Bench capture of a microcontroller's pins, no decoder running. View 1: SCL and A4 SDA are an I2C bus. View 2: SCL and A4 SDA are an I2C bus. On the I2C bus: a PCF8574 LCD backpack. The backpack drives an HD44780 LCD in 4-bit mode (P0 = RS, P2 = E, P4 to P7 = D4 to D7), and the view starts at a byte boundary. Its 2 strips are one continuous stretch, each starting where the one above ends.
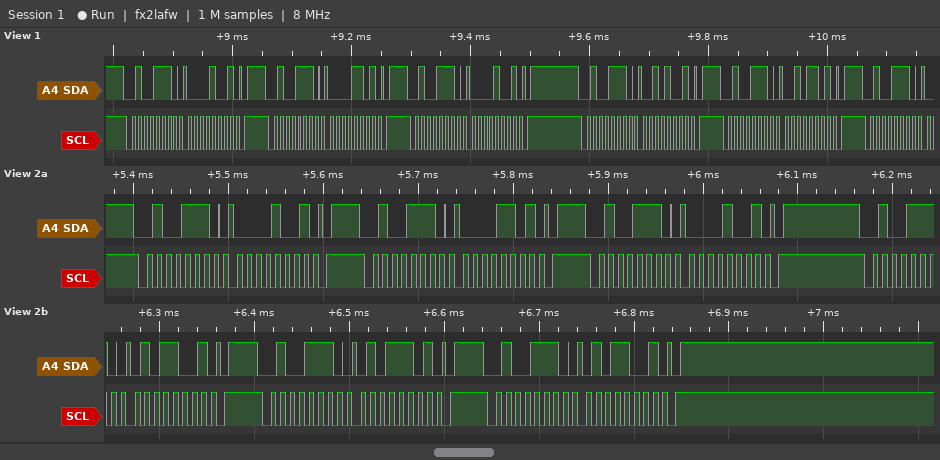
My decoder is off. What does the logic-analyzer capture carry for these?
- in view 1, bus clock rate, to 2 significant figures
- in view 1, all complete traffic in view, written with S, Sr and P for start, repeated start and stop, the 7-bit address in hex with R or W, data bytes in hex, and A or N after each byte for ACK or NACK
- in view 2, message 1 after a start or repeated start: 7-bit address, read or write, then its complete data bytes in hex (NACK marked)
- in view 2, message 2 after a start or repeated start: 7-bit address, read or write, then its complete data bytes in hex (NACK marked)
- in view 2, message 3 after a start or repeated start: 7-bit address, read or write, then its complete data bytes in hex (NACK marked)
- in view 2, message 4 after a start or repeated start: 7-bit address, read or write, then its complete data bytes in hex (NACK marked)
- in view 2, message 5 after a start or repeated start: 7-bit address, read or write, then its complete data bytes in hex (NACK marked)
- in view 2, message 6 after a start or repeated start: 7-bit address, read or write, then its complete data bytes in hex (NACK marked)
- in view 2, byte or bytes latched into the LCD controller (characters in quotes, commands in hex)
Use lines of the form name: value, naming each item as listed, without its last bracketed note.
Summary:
in view 1, bus clock rate, to 2 significant figures: 100 kHz
in view 1, all complete traffic in view, written with S, Sr and P for start, repeated start and stop, the 7-bit address in hex with R or W, data bytes in hex, and A or N after each byte for ACK or NACK: S 27W A 09 A P S 27W A 0D A P S 27W A 09 A P S 27W A 29 A P S 27W A 2D A P S 27W A
in view 2, message 1 after a start or repeated start: 7-bit address, read or write, then its complete data bytes in hex: 0x27 write: 09
in view 2, message 2 after a start or repeated start: 7-bit address, read or write, then its complete data bytes in hex: 0x27 write: 0D
in view 2, message 3 after a start or repeated start: 7-bit address, read or write, then its complete data bytes in hex: 0x27 write: 09
in view 2, message 4 after a start or repeated start: 7-bit address, read or write, then its complete data bytes in hex: 0x27 write: 59
in view 2, message 5 after a start or repeated start: 7-bit address, read or write, then its complete data bytes in hex: 0x27 write: 5D
in view 2, message 6 after a start or repeated start: 7-bit address, read or write, then its complete data bytes in hex: 0x27 write: 59
in view 2, byte or bytes latched into the LCD controller: data 0x05
